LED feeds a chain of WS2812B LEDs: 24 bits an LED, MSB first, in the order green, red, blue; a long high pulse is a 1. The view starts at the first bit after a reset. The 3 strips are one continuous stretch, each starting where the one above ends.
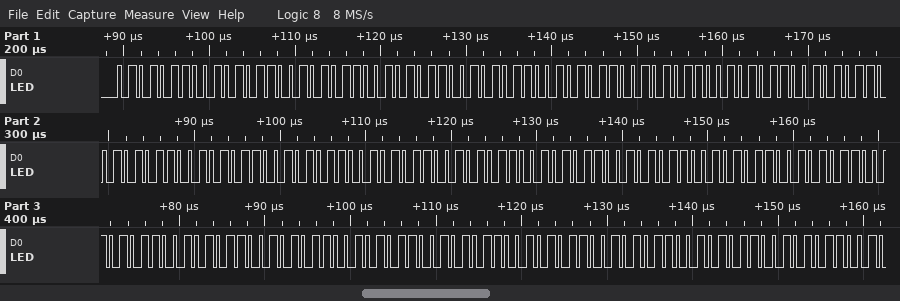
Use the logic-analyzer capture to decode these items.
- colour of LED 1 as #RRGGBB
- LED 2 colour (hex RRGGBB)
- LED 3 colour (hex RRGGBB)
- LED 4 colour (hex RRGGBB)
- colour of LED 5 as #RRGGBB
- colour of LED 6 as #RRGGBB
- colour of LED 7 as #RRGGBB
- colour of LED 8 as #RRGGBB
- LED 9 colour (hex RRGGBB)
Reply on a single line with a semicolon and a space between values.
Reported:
#565656; #565656; #565656; #565656; #565656; #565656; #565656; #565656; #565656
